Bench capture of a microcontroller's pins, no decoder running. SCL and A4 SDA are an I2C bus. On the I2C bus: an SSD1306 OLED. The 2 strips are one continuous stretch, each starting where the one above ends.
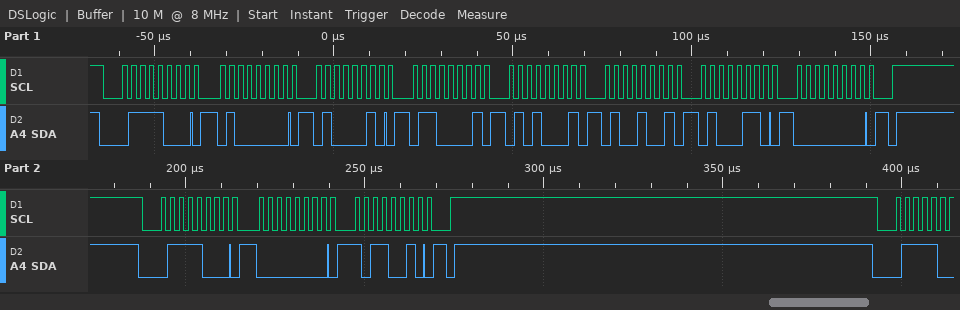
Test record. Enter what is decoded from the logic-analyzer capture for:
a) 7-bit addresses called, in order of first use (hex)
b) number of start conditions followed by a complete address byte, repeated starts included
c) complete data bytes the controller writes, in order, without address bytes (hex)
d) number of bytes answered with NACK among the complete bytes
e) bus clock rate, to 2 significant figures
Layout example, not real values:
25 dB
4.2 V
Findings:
0x3C
2
40 42 61 51 49 46 00 00 B2
0
400 kHz
